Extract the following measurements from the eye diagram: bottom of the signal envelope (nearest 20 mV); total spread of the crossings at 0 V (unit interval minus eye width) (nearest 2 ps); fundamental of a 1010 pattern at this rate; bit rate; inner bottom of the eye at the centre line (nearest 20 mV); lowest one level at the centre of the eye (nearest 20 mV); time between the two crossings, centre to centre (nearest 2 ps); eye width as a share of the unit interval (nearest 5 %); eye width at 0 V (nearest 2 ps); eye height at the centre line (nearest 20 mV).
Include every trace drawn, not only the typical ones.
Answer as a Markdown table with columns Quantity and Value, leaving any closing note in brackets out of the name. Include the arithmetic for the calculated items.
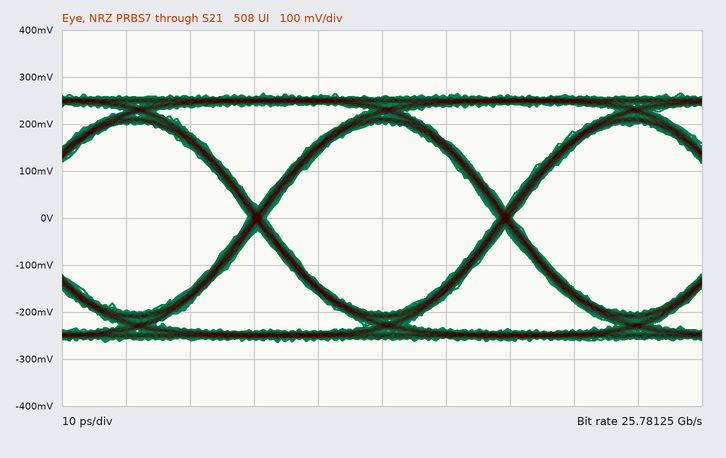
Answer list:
| Quantity | Value |
|---|---|
| bottom of the signal envelope | -260 mV |
| total spread of the crossings at 0 V (unit interval minus eye width) | 2 ps |
| fundamental of a 1010 pattern at this rate | 12.89062 GHz |
| bit rate | 25.78125 Gb/s |
| inner bottom of the eye at the centre line | -200 mV |
| lowest one level at the centre of the eye | 200 mV |
| time between the two crossings, centre to centre | 38 ps |
| eye width as a share of the unit interval | 36 ps / 38 ps ≈ 95 % |
| eye width at 0 V | 36 ps |
| eye height at the centre line | 400 mV |
